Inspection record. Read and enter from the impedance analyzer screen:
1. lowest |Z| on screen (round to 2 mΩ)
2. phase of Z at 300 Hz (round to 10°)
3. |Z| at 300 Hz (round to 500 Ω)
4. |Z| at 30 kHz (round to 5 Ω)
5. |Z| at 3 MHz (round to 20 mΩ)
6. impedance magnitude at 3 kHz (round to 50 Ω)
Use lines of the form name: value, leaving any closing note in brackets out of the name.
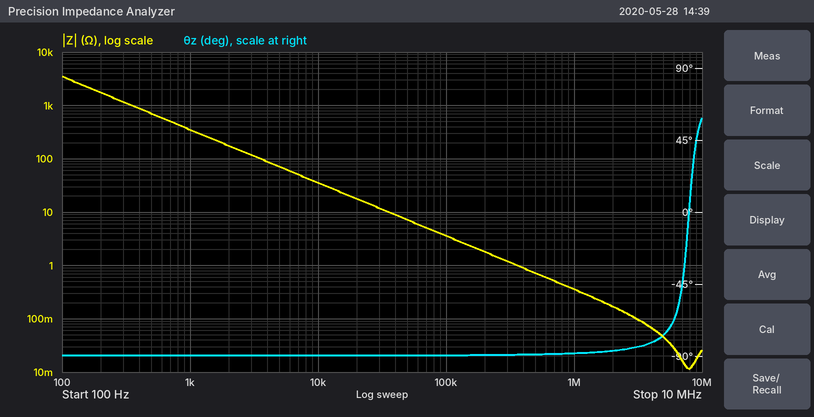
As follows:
lowest |Z| on screen: 12 mΩ
phase of Z at 300 Hz: -90°
|Z| at 300 Hz: 1.0 kΩ
|Z| at 30 kHz: 10 Ω
|Z| at 3 MHz: 100 mΩ
impedance magnitude at 3 kHz: 100 Ω
